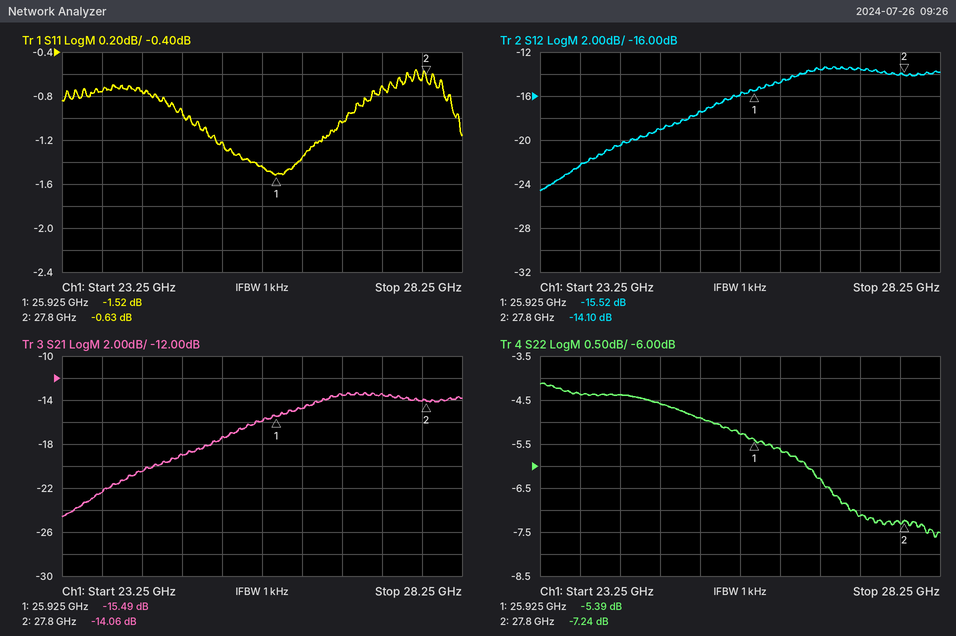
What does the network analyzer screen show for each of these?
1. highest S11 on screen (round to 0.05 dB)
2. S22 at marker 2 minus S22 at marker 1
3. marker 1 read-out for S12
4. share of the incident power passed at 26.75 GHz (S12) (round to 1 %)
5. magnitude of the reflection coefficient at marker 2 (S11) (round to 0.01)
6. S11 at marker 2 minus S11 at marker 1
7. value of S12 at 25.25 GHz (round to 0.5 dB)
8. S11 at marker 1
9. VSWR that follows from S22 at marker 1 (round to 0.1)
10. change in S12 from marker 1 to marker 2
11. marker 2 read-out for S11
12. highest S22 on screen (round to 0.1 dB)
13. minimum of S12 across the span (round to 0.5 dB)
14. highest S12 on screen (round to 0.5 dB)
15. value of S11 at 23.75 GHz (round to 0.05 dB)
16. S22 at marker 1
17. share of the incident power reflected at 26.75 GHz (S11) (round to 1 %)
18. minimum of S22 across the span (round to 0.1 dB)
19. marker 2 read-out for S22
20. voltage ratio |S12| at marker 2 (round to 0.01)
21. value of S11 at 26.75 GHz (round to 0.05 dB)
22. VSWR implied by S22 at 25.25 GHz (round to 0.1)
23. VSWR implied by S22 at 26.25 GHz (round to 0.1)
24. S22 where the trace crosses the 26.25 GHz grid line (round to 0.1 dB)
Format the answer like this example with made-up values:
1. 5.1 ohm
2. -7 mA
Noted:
1. -0.55 dB
2. -1.85 dB
3. -15.52 dB
4. 4 %
5. 0.93
6. 0.89 dB
7. -17.5 dB
8. -1.52 dB
9. 3.3
10. 1.42 dB
11. -0.63 dB
12. -4.1 dB
13. -24.5 dB
14. -13.5 dB
15. -0.75 dB
16. -5.39 dB
17. 79 %
18. -7.6 dB
19. -7.24 dB
20. 0.20
21. -1.05 dB
22. 3.6
23. 3.2
24. -5.6 dB
